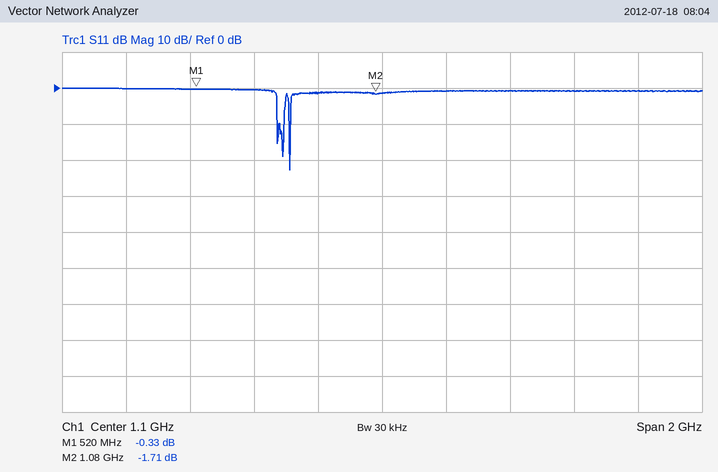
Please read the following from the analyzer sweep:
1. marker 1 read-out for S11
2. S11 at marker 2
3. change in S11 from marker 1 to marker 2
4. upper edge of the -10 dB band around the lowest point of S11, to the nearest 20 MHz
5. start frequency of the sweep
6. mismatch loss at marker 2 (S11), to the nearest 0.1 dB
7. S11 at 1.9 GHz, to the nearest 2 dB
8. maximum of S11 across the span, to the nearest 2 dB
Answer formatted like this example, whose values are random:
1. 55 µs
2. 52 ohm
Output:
1. -0.33 dB
2. -1.71 dB
3. -1.38 dB
4. 820 MHz
5. 100 MHz
6. 4.9 dB
7. 0 dB
8. 0 dB
